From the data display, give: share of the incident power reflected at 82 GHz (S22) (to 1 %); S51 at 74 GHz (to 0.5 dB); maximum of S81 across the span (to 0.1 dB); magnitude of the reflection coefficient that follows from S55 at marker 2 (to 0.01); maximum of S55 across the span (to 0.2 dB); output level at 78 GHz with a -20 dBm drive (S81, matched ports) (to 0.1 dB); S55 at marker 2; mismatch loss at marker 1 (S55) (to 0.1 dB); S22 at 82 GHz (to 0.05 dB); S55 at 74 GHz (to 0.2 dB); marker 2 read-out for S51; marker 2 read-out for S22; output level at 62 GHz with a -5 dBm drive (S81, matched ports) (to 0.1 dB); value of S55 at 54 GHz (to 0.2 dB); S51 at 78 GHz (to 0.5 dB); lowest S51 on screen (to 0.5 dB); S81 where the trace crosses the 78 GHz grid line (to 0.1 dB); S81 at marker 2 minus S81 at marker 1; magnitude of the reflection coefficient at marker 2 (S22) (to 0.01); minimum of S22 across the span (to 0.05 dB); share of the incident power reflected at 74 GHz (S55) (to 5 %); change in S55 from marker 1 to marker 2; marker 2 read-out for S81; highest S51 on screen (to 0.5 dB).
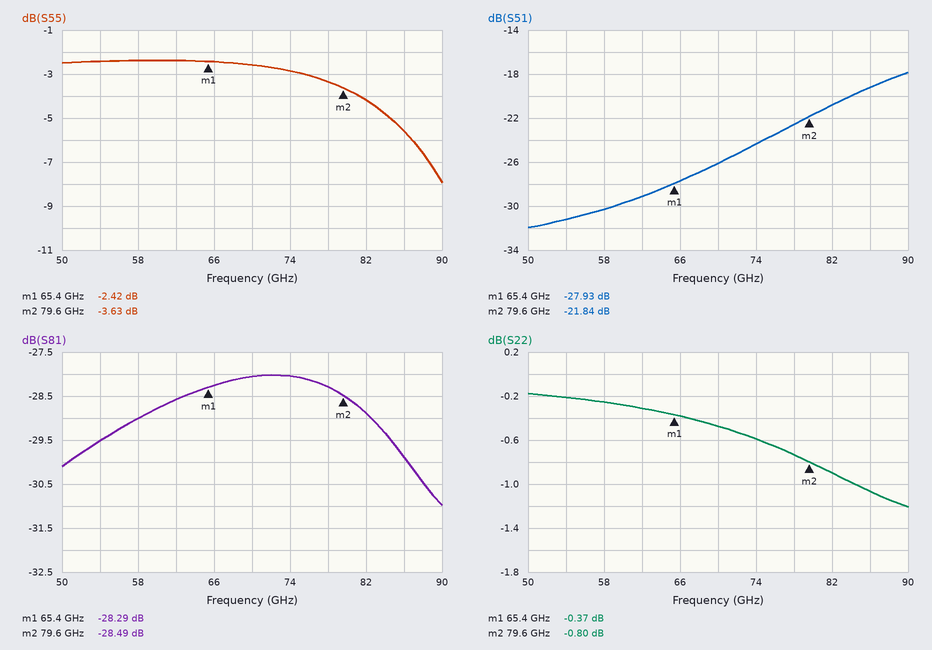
81 %
-24.5 dB
-28.0 dB
0.66
-2.4 dB
-48.3 dBm
-3.63 dB
3.7 dB
-0.90 dB
-2.8 dB
-21.84 dB
-0.80 dB
-33.6 dBm
-2.4 dB
-22.5 dB
-32.0 dB
-28.3 dB
-0.20 dB
0.91
-1.20 dB
50 %
-1.21 dB
-28.49 dB
-18.0 dB
